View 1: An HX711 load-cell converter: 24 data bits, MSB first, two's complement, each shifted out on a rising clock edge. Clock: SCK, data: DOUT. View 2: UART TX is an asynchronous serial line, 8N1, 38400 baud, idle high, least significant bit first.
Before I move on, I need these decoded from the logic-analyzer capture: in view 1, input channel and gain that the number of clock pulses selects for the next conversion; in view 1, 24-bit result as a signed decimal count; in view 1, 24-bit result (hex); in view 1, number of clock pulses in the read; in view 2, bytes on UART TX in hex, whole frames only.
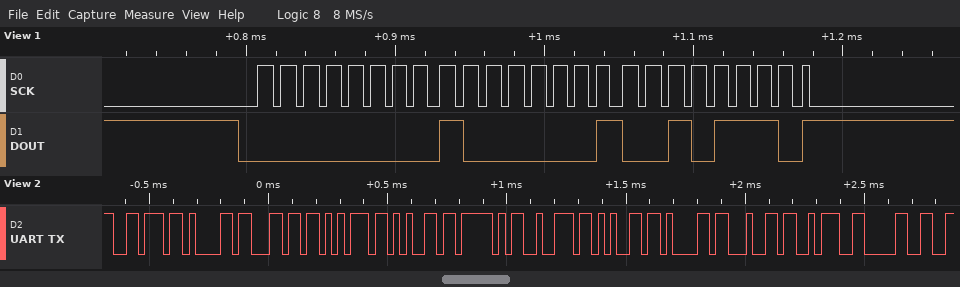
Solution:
channel A, gain 128
33070
0x00812E
25
76 61 6C 75 65 5F 72 65 61 64 3A 30
